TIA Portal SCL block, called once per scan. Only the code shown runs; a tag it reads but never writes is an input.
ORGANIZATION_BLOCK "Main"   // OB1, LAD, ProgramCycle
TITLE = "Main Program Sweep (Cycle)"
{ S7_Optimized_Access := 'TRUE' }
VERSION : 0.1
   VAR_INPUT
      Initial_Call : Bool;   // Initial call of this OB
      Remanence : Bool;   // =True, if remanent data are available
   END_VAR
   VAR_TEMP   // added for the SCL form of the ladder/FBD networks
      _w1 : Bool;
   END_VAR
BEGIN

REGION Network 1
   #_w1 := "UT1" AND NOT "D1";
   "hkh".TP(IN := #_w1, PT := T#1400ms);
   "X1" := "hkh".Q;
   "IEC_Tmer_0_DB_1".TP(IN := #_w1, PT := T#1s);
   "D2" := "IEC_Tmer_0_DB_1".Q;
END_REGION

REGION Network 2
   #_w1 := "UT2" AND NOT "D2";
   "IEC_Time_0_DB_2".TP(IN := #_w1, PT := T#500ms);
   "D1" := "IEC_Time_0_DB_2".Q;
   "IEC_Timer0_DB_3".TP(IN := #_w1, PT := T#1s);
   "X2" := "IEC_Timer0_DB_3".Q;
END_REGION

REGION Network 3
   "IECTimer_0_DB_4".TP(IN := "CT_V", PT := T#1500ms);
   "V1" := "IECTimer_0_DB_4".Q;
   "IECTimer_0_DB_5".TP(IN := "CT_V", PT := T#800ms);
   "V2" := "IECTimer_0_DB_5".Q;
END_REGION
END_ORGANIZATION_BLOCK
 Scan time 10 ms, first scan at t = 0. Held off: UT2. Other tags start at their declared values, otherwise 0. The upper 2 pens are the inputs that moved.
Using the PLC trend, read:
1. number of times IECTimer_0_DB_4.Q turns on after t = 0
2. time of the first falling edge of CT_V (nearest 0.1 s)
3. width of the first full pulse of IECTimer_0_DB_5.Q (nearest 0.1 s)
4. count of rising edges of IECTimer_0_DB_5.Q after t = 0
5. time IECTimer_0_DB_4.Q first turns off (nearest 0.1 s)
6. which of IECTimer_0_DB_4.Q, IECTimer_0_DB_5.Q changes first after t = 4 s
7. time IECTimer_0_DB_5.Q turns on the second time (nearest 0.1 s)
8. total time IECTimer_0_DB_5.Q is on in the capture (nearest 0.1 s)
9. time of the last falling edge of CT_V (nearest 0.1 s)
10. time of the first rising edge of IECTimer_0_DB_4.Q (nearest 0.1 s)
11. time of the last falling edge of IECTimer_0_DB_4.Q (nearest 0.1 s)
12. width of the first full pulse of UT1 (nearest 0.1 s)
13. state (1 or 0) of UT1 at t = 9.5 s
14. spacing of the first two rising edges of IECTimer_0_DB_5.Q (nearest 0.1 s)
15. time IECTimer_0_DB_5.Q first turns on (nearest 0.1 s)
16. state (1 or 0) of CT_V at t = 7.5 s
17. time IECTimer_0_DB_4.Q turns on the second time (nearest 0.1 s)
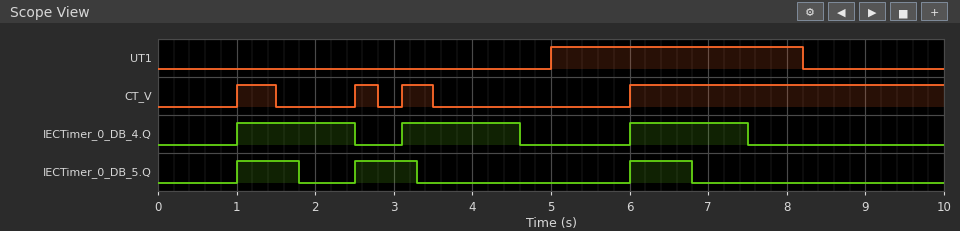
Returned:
3
1.5 s
0.8 s
3
2.5 s
IECTimer_0_DB_4.Q
2.5 s
2.4 s
3.5 s
1.0 s
7.5 s
3.2 s
0
1.5 s
1.0 s
1
3.1 s
